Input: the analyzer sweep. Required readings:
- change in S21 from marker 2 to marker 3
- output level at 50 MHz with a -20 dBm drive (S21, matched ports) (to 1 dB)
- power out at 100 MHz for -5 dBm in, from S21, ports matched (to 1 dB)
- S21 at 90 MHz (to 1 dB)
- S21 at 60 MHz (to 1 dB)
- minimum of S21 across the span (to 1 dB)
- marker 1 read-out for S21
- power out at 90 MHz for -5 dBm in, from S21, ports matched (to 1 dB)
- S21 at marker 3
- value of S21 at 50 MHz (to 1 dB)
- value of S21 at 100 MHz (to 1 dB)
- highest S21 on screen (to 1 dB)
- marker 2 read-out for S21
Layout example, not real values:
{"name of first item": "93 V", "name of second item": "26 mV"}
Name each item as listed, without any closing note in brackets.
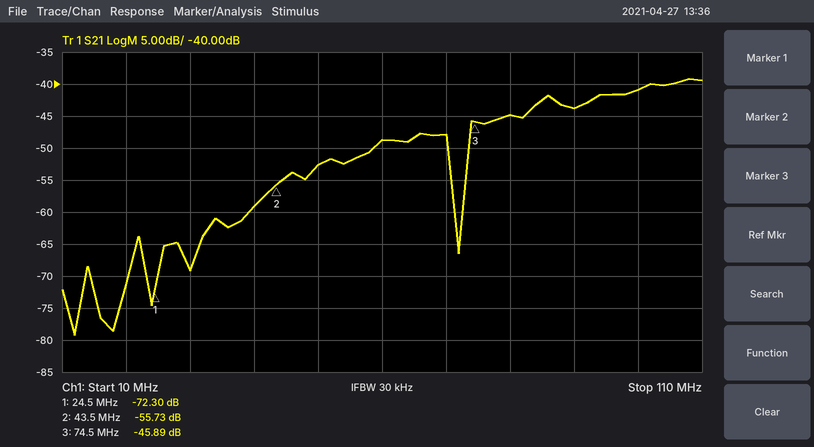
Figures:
{"change in S21 from marker 2 to marker 3": "9.84 dB", "output level at 50 MHz with a -20 dBm drive (S21, matched ports)": "-73 dBm", "power out at 100 MHz for -5 dBm in, from S21, ports matched": "-46 dBm", "S21 at 90 MHz": "-44 dB", "S21 at 60 MHz": "-49 dB", "minimum of S21 across the span": "-79 dB", "marker 1 read-out for S21": "-72.30 dB", "power out at 90 MHz for -5 dBm in, from S21, ports matched": "-49 dBm", "S21 at marker 3": "-45.89 dB", "value of S21 at 50 MHz": "-53 dB", "value of S21 at 100 MHz": "-41 dB", "highest S21 on screen": "-39 dB", "marker 2 read-out for S21": "-55.73 dB"}
